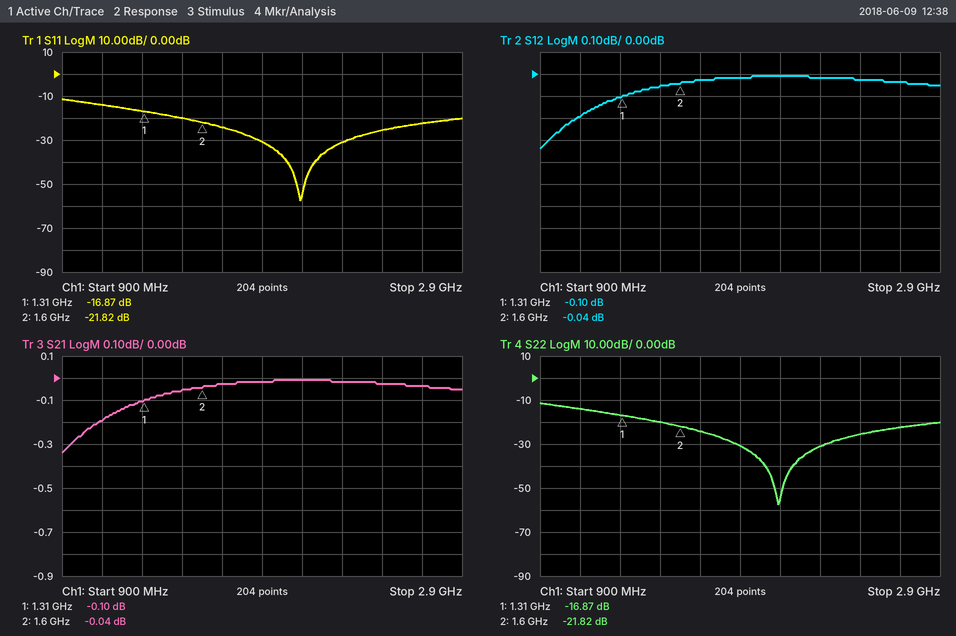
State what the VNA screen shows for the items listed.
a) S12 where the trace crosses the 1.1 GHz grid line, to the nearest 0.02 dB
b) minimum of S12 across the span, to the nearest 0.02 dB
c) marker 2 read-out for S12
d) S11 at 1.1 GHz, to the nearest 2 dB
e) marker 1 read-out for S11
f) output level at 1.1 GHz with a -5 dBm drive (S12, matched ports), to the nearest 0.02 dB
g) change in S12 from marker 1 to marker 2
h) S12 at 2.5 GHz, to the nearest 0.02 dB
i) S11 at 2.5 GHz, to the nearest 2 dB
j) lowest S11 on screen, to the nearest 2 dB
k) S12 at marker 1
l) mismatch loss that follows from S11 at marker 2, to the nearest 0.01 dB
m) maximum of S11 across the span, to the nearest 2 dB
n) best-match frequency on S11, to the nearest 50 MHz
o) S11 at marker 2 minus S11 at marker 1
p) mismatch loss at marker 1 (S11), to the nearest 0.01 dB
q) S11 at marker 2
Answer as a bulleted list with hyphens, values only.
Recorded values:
- -0.20 dB
- -0.34 dB
- -0.04 dB
- -14 dB
- -16.87 dB
- -5.20 dBm
- 0.06 dB
- -0.02 dB
- -26 dB
- -58 dB
- -0.10 dB
- 0.03 dB
- -12 dB
- 2.10 GHz
- -4.95 dB
- 0.09 dB
- -21.82 dB
